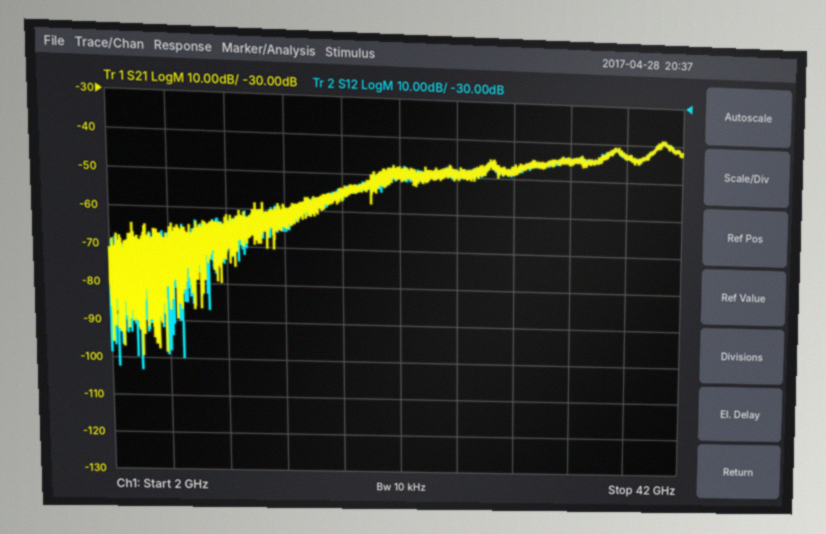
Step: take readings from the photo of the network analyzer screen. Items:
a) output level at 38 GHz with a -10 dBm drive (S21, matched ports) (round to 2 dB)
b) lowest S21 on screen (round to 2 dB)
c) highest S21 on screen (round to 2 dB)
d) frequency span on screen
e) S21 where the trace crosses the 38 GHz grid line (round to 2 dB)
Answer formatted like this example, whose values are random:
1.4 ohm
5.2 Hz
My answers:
-54 dBm
-100 dB
-38 dB
40 GHz
-44 dB
